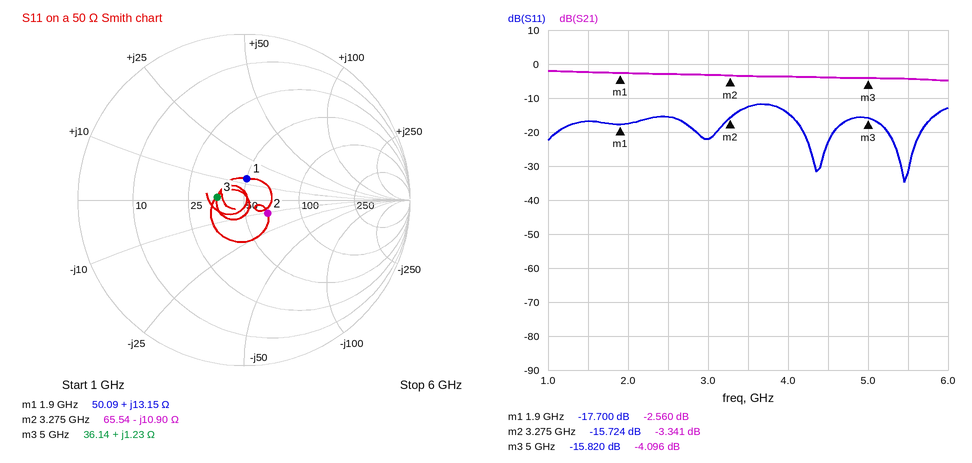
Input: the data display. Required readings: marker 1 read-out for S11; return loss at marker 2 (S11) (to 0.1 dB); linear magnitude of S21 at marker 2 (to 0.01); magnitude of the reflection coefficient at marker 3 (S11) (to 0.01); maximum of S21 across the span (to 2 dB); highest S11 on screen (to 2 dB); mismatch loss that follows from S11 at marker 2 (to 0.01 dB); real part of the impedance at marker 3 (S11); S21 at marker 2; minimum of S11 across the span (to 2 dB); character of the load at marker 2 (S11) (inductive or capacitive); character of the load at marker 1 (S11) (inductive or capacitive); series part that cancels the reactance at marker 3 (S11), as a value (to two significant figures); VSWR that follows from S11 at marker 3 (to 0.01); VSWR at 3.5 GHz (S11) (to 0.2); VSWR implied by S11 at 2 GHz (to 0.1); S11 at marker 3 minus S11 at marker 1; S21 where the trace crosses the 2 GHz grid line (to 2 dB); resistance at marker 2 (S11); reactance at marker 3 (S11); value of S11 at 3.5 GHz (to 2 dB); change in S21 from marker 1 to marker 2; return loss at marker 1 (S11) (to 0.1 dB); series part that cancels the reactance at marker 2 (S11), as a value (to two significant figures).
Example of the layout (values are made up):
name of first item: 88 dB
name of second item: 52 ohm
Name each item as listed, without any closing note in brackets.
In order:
marker 1 read-out for S11: -17.700 dB
return loss at marker 2 (S11): 15.7 dB
linear magnitude of S21 at marker 2: 0.68
magnitude of the reflection coefficient at marker 3 (S11): 0.16
maximum of S21 across the span: -2 dB
highest S11 on screen: -12 dB
mismatch loss that follows from S11 at marker 2: 0.12 dB
real part of the impedance at marker 3: 36.14 Ω
S21 at marker 2: -3.341 dB
minimum of S11 across the span: -34 dB
character of the load at marker 2 (S11): capacitive
character of the load at marker 1 (S11): inductive
series part that cancels the reactance at marker 3 (S11), as a value: 26 pF
VSWR that follows from S11 at marker 3: 1.39
VSWR at 3.5 GHz (S11): 1.6
VSWR implied by S11 at 2 GHz: 1.3
S11 at marker 3 minus S11 at marker 1: 1.880 dB
S21 where the trace crosses the 2 GHz grid line: -2 dB
resistance at marker 2: 65.54 Ω
reactance at marker 3: +1.23 Ω
value of S11 at 3.5 GHz: -12 dB
change in S21 from marker 1 to marker 2: -0.781 dB
return loss at marker 1 (S11): 17.7 dB
series part that cancels the reactance at marker 2 (S11), as a value: 530 pH
